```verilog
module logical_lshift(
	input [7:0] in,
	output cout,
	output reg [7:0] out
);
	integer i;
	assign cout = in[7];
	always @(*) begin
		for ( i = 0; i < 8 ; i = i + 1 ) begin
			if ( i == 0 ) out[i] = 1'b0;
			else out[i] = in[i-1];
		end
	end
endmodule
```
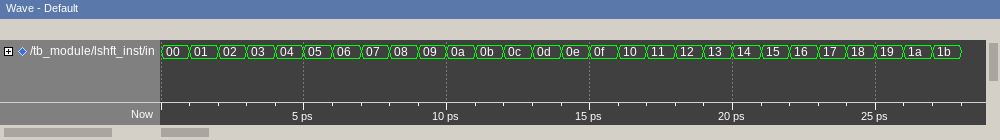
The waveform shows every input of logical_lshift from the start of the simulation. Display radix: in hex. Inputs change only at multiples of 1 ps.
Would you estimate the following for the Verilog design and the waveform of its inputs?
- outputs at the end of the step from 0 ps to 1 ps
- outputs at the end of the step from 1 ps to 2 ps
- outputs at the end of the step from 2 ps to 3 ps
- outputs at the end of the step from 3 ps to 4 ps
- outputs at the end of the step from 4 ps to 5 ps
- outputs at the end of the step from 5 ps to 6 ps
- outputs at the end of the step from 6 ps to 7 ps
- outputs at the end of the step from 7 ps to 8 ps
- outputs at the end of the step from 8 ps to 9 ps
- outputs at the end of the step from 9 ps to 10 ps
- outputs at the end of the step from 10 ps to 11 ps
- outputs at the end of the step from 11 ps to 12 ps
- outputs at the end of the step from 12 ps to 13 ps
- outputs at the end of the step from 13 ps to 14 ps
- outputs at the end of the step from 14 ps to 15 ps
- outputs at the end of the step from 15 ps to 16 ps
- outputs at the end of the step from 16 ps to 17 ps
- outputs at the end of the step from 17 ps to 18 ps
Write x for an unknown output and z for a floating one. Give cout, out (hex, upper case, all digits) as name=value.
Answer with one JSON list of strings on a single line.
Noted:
["cout=0, out=00", "cout=0, out=02", "cout=0, out=04", "cout=0, out=06", "cout=0, out=08", "cout=0, out=0A", "cout=0, out=0C", "cout=0, out=0E", "cout=0, out=10", "cout=0, out=12", "cout=0, out=14", "cout=0, out=16", "cout=0, out=18", "cout=0, out=1A", "cout=0, out=1C", "cout=0, out=1E", "cout=0, out=20", "cout=0, out=22"]
